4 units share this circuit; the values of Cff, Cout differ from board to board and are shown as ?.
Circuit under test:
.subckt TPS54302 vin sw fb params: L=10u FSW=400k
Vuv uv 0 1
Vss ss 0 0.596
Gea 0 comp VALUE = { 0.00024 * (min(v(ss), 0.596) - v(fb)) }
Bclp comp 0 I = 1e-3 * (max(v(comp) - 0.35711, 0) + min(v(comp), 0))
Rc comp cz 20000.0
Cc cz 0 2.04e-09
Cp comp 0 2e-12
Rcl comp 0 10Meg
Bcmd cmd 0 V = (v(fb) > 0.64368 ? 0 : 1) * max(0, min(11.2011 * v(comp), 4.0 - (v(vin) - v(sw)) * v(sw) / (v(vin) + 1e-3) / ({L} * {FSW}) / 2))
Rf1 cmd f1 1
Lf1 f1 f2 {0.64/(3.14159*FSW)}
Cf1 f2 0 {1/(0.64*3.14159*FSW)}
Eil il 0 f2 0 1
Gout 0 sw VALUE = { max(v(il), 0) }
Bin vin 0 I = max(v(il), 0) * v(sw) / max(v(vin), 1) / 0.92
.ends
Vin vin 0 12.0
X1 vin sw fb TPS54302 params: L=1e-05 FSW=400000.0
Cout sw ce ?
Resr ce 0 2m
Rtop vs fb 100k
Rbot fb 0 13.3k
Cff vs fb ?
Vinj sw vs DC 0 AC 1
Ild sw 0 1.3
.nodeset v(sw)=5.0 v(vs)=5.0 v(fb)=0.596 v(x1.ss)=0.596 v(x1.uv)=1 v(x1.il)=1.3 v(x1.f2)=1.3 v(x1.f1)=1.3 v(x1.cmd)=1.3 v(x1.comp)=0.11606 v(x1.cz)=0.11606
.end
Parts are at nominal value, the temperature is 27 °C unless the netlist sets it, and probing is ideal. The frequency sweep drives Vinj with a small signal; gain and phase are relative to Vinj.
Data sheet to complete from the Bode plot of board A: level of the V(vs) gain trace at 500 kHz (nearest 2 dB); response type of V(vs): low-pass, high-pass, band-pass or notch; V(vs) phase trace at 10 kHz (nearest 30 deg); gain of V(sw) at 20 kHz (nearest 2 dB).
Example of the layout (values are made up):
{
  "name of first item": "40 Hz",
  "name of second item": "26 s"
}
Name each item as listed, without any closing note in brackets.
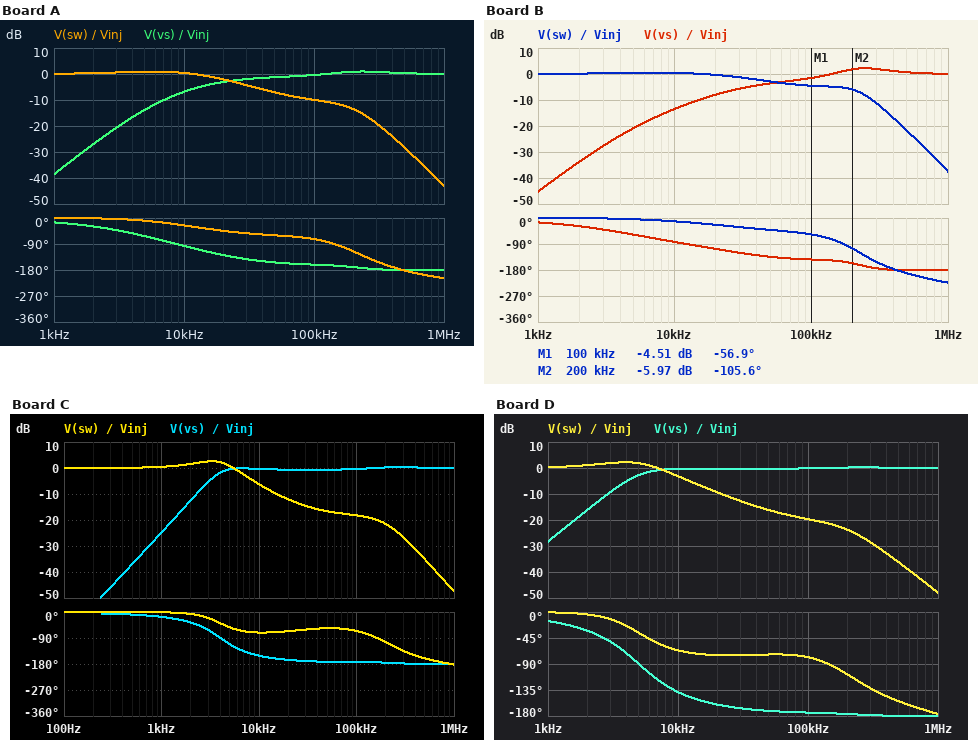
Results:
{
  "level of the V(vs) gain trace at 500 kHz": "0 dB",
  "response type of V(vs): low-pass, high-pass, band-pass or notch": "high-pass",
  "V(vs) phase trace at 10 kHz": "-90 deg",
  "gain of V(sw) at 20 kHz": "-2 dB"
}
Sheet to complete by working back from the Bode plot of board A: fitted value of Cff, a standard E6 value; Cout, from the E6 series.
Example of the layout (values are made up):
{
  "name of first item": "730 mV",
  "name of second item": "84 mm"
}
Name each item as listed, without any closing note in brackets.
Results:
{
  "fitted value of Cff, a standard E6 value": "22 pF",
  "Cout, from the E6 series": "47 µF"
}
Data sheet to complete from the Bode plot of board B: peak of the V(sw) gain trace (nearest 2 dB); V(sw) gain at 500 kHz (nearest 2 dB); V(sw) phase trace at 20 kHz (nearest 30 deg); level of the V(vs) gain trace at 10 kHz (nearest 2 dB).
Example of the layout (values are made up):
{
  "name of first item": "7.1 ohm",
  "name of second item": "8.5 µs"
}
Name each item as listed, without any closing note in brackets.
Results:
{
  "peak of the V(sw) gain trace": "0 dB",
  "V(sw) gain at 500 kHz": "-22 dB",
  "V(sw) phase trace at 20 kHz": "-30 deg",
  "level of the V(vs) gain trace at 10 kHz": "-14 dB"
}
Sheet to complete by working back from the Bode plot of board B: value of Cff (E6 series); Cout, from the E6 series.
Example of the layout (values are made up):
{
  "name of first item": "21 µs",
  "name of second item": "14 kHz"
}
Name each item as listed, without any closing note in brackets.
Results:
{
  "value of Cff": "22 pF",
  "Cout, from the E6 series": "22 µF"
}
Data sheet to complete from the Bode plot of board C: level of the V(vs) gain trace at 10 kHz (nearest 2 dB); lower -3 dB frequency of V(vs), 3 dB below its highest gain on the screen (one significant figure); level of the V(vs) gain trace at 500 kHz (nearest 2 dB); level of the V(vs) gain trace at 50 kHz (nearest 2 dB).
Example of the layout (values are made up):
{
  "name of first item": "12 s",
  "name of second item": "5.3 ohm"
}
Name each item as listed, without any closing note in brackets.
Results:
{
  "level of the V(vs) gain trace at 10 kHz": "0 dB",
  "lower -3 dB frequency of V(vs), 3 dB below its highest gain on the screen": "4 kHz",
  "level of the V(vs) gain trace at 500 kHz": "0 dB",
  "level of the V(vs) gain trace at 50 kHz": "0 dB"
}
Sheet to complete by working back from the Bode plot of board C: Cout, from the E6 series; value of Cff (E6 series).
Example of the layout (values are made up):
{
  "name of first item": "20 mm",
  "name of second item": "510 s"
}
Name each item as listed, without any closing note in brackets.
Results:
{
  "Cout, from the E6 series": "220 µF",
  "value of Cff": "47 pF"
}
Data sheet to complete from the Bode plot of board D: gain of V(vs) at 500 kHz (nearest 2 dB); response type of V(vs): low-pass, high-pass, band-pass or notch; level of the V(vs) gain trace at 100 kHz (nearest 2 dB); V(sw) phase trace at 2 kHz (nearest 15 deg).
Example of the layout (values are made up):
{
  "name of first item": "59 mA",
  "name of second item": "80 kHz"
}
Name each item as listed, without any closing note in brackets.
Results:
{
  "gain of V(vs) at 500 kHz": "0 dB",
  "response type of V(vs): low-pass, high-pass, band-pass or notch": "high-pass",
  "level of the V(vs) gain trace at 100 kHz": "0 dB",
  "V(sw) phase trace at 2 kHz": "0 deg"
}
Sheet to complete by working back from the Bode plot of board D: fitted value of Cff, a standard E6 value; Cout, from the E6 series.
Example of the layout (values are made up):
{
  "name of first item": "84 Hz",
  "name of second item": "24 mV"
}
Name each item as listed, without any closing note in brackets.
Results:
{
  "fitted value of Cff, a standard E6 value": "22 pF",
  "Cout, from the E6 series": "150 µF"
}
